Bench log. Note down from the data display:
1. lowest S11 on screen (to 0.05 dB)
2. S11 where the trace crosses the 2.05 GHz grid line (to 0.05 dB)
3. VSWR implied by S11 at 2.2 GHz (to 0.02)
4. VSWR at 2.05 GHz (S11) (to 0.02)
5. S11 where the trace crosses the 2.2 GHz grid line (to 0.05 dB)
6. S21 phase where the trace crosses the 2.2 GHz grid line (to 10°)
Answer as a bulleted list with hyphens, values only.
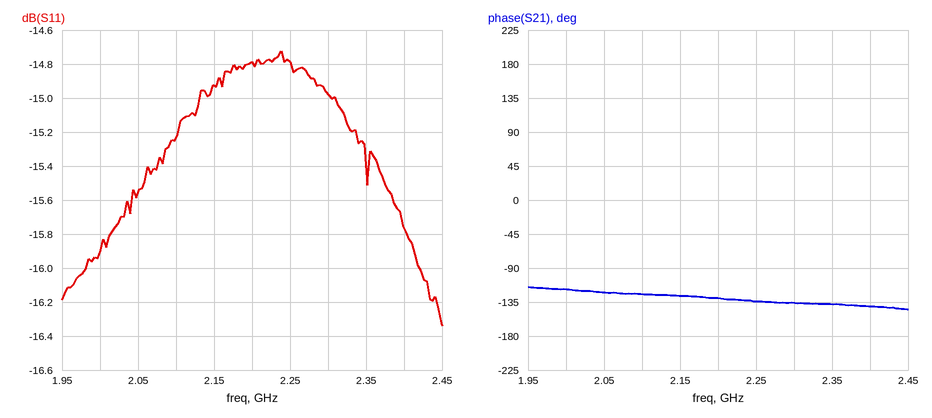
- -16.35 dB
- -15.55 dB
- 1.44
- 1.40
- -14.80 dB
- -130°
